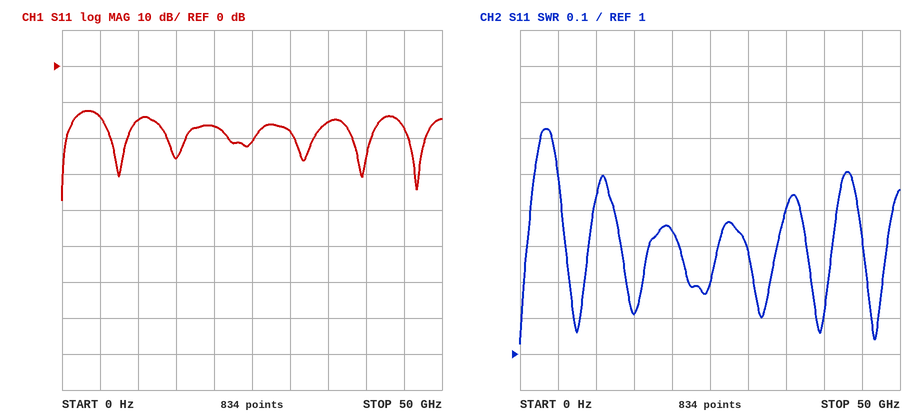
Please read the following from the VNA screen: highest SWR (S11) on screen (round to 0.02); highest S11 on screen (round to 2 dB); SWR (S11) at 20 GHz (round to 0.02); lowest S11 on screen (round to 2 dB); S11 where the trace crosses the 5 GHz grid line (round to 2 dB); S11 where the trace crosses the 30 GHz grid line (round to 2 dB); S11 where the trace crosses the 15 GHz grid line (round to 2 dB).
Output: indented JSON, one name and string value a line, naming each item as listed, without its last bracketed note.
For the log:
{
  "highest SWR (S11) on screen": "1.62",
  "highest S11 on screen": "-12 dB",
  "SWR (S11) at 20 GHz": "1.34",
  "lowest S11 on screen": "-38 dB",
  "S11 where the trace crosses the 5 GHz grid line": "-14 dB",
  "S11 where the trace crosses the 30 GHz grid line": "-18 dB",
  "S11 where the trace crosses the 15 GHz grid line": "-26 dB"
}
